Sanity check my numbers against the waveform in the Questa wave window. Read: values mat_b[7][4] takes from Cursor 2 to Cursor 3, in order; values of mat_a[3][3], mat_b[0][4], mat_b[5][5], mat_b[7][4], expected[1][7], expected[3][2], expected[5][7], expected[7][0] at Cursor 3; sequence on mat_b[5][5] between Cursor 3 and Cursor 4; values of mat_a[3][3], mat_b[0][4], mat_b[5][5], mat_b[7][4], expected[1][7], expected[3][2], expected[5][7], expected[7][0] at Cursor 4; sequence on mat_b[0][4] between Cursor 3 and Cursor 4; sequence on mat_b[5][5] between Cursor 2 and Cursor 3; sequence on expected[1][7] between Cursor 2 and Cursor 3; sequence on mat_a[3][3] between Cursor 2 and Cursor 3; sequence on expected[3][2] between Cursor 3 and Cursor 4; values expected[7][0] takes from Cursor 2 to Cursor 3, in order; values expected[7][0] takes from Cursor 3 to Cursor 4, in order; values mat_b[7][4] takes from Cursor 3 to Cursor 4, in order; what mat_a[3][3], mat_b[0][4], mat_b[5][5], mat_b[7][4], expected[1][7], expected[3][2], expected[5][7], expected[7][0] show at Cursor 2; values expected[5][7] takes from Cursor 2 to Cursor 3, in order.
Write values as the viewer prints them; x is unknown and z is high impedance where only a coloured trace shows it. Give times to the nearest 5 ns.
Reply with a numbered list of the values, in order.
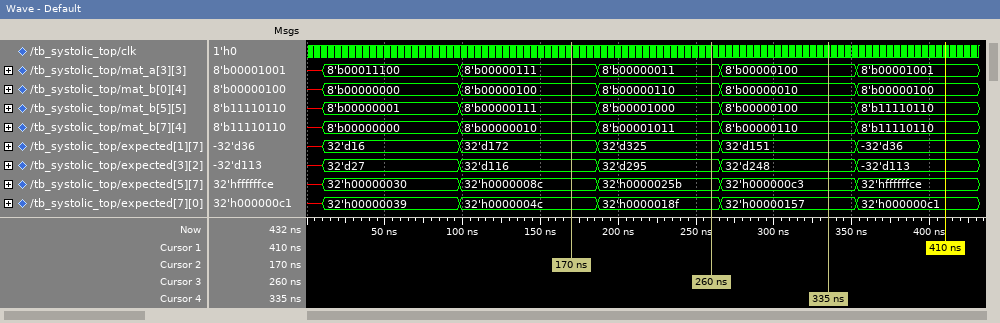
1. 8'b00000010, 8'b00001011
2. mat_a[3][3]=8'b00000011, mat_b[0][4]=8'b00000110, mat_b[5][5]=8'b00001000, mat_b[7][4]=8'b00001011, expected[1][7]=32'd325, expected[3][2]=32'd295, expected[5][7]=32'h0000025b, expected[7][0]=32'h0000018f
3. 8'b00001000, 8'b00000100
4. mat_a[3][3]=8'b00000100, mat_b[0][4]=8'b00000010, mat_b[5][5]=8'b00000100, mat_b[7][4]=8'b00000110, expected[1][7]=32'd151, expected[3][2]=32'd248, expected[5][7]=32'h000000c3, expected[7][0]=32'h00000157
5. 8'b00000110, 8'b00000010
6. 8'b00000111, 8'b00001000
7. 32'd172, 32'd325
8. 8'b00000111, 8'b00000011
9. 32'd295, 32'd248
10. 32'h0000004c, 32'h0000018f
11. 32'h0000018f, 32'h00000157
12. 8'b00001011, 8'b00000110
13. mat_a[3][3]=8'b00000111, mat_b[0][4]=8'b00000100, mat_b[5][5]=8'b00000111, mat_b[7][4]=8'b00000010, expected[1][7]=32'd172, expected[3][2]=32'd116, expected[5][7]=32'h0000008c, expected[7][0]=32'h0000004c
14. 32'h0000008c, 32'h0000025b
